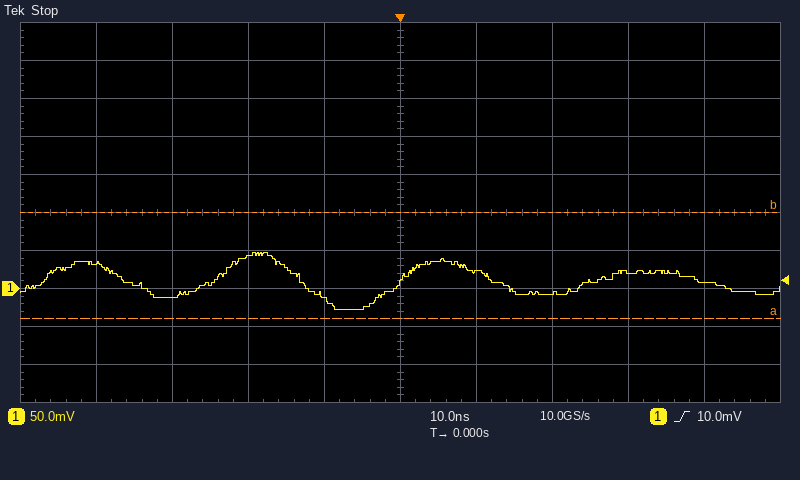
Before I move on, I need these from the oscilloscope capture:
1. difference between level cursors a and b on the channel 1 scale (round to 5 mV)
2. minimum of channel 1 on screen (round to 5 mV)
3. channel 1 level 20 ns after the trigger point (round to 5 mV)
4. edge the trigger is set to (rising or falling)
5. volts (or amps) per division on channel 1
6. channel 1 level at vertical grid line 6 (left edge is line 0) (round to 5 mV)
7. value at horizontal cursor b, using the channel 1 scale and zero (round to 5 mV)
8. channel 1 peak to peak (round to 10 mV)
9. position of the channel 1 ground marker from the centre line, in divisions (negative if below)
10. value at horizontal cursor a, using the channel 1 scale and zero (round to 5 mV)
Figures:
140 mV
-30 mV
-5 mV
rising
50 mV
20 mV
100 mV
80 mV
-2.0 div
-40 mV
